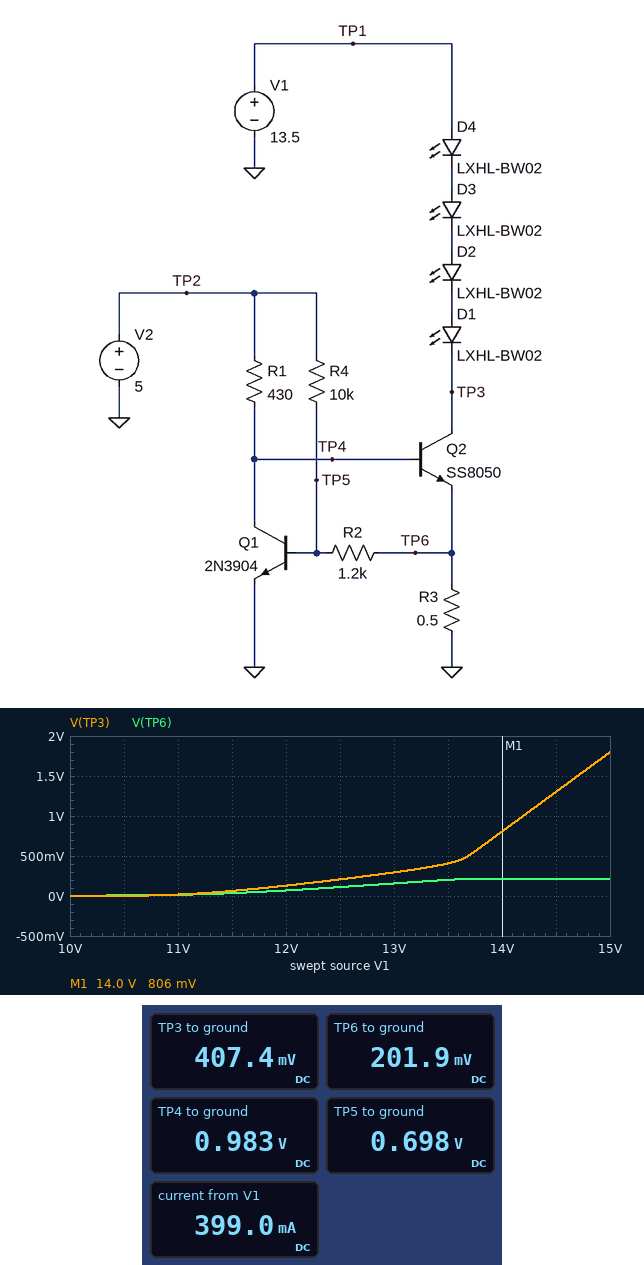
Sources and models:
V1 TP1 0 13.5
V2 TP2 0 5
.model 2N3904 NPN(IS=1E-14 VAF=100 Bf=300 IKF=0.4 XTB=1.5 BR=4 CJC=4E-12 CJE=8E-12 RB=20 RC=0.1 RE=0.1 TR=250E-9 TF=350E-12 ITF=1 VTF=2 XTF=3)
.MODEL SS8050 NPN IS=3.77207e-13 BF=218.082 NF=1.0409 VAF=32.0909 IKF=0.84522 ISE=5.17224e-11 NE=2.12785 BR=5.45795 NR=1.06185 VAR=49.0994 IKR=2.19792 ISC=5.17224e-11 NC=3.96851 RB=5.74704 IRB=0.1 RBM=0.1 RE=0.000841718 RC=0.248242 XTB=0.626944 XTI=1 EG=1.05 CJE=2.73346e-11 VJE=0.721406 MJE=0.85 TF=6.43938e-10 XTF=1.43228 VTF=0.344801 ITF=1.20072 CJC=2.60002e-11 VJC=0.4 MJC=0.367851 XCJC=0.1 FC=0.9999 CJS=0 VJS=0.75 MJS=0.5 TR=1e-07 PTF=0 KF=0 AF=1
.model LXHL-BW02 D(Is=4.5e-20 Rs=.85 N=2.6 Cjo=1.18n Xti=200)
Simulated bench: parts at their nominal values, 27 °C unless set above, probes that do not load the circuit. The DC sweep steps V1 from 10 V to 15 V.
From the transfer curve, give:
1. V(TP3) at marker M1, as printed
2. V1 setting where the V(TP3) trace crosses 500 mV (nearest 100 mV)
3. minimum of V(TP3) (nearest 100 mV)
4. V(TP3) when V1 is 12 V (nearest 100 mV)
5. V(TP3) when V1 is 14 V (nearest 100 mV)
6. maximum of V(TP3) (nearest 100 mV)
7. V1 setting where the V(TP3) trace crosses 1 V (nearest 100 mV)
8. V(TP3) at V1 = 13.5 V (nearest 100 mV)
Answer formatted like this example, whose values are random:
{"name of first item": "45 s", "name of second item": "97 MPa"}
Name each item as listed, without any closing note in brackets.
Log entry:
{"V(TP3) at marker M1, as printed": "806 mV", "V1 setting where the V(TP3) trace crosses 500 mV": "13.7 V", "minimum of V(TP3)": "0 V", "V(TP3) when V1 is 12 V": "100 mV", "V(TP3) when V1 is 14 V": "800 mV", "maximum of V(TP3)": "1.8 V", "V1 setting where the V(TP3) trace crosses 1 V": "14.2 V", "V(TP3) at V1 = 13.5 V": "400 mV"}
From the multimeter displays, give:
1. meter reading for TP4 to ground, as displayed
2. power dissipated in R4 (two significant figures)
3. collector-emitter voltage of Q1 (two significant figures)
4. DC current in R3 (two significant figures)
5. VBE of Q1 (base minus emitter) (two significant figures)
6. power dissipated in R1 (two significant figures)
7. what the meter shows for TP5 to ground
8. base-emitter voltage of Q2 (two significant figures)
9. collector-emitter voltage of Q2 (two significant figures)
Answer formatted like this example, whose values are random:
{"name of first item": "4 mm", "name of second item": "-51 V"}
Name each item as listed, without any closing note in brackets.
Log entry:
{"meter reading for TP4 to ground, as displayed": "0.983 V", "power dissipated in R4": "1.9 mW", "collector-emitter voltage of Q1": "980 mV", "DC current in R3": "400 mA", "VBE of Q1 (base minus emitter)": "700 mV", "power dissipated in R1": "38 mW", "what the meter shows for TP5 to ground": "0.698 V", "base-emitter voltage of Q2": "780 mV", "collector-emitter voltage of Q2": "210 mV"}
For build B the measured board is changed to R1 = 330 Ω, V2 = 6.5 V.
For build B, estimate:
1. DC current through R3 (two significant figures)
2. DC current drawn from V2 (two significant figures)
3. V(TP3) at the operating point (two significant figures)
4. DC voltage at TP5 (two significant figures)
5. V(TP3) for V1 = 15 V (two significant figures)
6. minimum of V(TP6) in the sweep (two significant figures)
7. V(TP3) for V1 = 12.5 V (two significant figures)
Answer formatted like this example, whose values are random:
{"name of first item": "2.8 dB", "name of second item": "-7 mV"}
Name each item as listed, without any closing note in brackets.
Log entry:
{"DC current through R3": "210 mA", "DC current drawn from V2": "18 mA", "V(TP3) at the operating point": "1.2 V", "DC voltage at TP5": "730 mV", "V(TP3) for V1 = 15 V": "2.7 V", "minimum of V(TP6) in the sweep": "7.4 mV", "V(TP3) for V1 = 12.5 V": "270 mV"}
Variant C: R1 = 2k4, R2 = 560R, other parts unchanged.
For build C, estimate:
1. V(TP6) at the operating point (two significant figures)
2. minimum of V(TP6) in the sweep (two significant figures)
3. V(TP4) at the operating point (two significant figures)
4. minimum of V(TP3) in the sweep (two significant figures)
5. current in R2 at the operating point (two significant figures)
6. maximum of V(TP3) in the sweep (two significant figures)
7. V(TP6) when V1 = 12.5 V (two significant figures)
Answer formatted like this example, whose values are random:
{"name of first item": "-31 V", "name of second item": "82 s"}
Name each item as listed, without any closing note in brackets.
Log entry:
{"V(TP6) at the operating point": "140 mV", "minimum of V(TP6) in the sweep": "1.5 mV", "V(TP4) at the operating point": "890 mV", "minimum of V(TP3) in the sweep": "-5.1 mV", "current in R2 at the operating point": "460 µA", "maximum of V(TP3) in the sweep": "2.4 V", "V(TP6) when V1 = 12.5 V": "100 mV"}
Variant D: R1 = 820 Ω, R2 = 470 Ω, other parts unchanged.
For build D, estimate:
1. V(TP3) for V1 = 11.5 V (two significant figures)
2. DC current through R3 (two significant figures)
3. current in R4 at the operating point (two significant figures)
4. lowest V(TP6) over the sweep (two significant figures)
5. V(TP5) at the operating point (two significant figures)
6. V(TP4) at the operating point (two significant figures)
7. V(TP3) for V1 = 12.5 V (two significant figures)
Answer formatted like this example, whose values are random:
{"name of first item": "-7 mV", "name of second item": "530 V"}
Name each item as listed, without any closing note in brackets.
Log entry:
{"V(TP3) for V1 = 11.5 V": "71 mV", "DC current through R3": "410 mA", "current in R4 at the operating point": "460 µA", "lowest V(TP6) over the sweep": "3.2 mV", "V(TP5) at the operating point": "420 mV", "V(TP4) at the operating point": "990 mV", "V(TP3) for V1 = 12.5 V": "220 mV"}
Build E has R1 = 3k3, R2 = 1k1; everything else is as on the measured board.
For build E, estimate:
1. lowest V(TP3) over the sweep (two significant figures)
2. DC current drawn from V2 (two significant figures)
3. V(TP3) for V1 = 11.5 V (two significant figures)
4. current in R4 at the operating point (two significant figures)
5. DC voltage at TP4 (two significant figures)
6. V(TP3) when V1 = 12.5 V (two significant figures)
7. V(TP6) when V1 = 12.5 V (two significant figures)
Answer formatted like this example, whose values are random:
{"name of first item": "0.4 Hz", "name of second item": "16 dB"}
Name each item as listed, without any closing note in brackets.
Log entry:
{"lowest V(TP3) over the sweep": "-4.6 mV", "DC current drawn from V2": "1.7 mA", "V(TP3) for V1 = 11.5 V": "100 mV", "current in R4 at the operating point": "440 µA", "DC voltage at TP4": "840 mV", "V(TP3) when V1 = 12.5 V": "310 mV", "V(TP6) when V1 = 12.5 V": "96 mV"}
